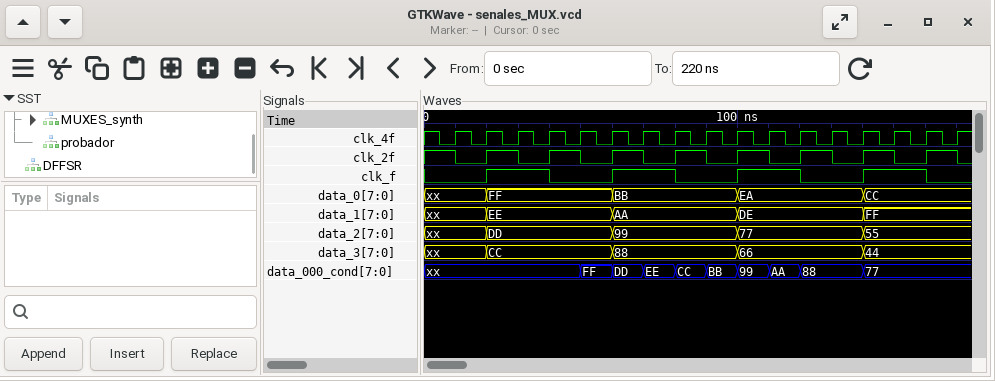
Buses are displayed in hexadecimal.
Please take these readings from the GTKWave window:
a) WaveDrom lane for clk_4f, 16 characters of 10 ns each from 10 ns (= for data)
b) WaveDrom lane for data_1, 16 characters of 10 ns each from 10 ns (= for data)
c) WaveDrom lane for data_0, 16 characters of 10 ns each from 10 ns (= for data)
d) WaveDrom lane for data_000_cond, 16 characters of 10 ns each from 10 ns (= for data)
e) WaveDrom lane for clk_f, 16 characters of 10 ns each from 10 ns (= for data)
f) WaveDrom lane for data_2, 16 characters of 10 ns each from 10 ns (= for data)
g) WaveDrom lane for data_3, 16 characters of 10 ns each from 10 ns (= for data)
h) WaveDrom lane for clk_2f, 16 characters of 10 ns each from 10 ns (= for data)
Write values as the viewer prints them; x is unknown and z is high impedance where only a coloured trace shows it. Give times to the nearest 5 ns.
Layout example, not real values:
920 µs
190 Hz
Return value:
{name: 'clk_4f', wave: 'p...............'}
{name: 'data_1', wave: 'x=...=...=...=..', data: 'EE AA DE FF'}
{name: 'data_0', wave: 'x=...=...=...=..', data: 'FF BB EA CC'}
{name: 'data_000_cond', wave: 'x...========.=..', data: 'FF DD EE CC BB 99 AA 88 77'}
{name: 'clk_f', wave: '01.0.1.0.1.0.1.0'}
{name: 'data_2', wave: 'x=...=...=...=..', data: 'DD 99 77 55'}
{name: 'data_3', wave: 'x=...=...=...=..', data: 'CC 88 66 44'}
{name: 'clk_2f', wave: '0101010101010101'}
